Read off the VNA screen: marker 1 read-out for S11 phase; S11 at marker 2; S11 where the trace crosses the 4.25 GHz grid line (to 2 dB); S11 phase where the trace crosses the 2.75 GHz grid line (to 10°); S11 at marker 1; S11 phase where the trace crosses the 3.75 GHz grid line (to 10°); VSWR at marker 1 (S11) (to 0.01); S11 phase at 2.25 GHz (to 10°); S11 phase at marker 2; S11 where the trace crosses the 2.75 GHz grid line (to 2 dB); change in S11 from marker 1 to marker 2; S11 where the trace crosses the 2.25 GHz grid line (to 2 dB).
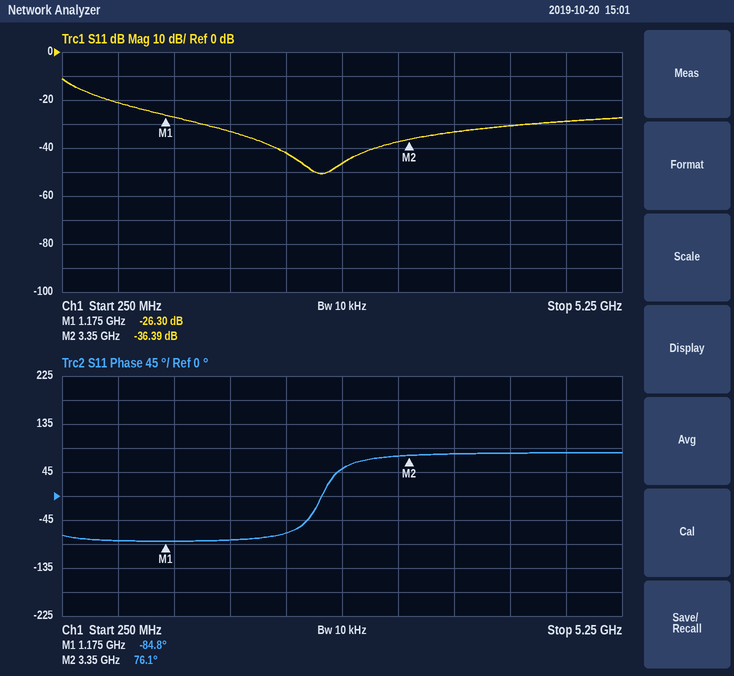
-84.8°
-36.39 dB
-30 dB
50°
-26.30 dB
80°
1.10
-70°
76.1°
-46 dB
-10.09 dB
-42 dB
